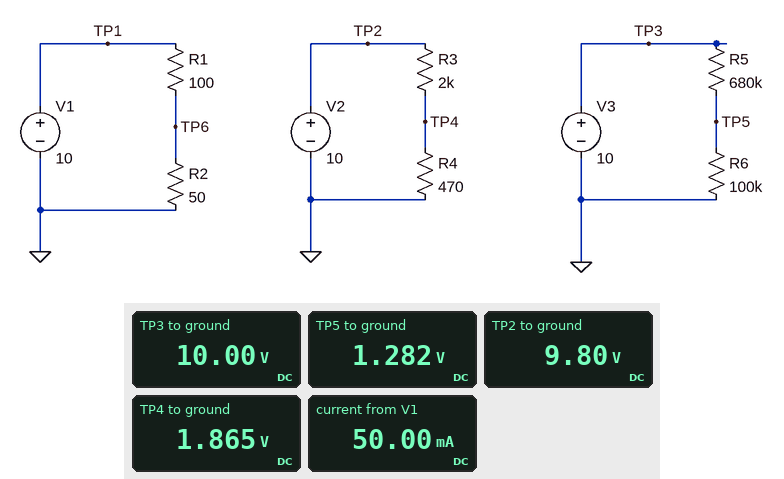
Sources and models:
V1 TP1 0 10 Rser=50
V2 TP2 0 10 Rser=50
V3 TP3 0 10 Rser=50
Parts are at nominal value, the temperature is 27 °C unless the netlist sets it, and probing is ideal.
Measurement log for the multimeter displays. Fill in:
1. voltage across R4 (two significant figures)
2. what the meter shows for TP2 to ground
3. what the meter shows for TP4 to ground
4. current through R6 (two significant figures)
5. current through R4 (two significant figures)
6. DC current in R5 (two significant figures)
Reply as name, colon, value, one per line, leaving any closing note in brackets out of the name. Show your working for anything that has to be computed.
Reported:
voltage across R4: 1.865 V = 1.9 V
what the meter shows for TP2 to ground: 9.80 V
what the meter shows for TP4 to ground: 1.865 V
current through R6: (1.282 V) / 100 kΩ = 13 µA
current through R4: (1.865 V) / 470 Ω = 4.0 mA
DC current in R5: (10 V - 1.282 V) / 680 kΩ = 13 µA
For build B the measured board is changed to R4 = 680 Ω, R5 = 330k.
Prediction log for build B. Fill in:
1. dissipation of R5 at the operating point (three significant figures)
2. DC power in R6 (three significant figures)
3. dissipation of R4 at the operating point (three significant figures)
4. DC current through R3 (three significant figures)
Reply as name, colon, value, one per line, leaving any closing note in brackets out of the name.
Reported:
dissipation of R5 at the operating point: 178 µW
DC power in R6: 54.1 µW
dissipation of R4 at the operating point: 9.12 mW
DC current through R3: 3.66 mA
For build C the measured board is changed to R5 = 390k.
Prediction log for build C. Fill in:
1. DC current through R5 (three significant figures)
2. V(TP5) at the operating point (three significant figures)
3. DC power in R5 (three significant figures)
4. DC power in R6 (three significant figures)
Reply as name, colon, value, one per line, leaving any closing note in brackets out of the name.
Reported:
DC current through R5: 20.4 µA
V(TP5) at the operating point: 2.04 V
DC power in R5: 162 µW
DC power in R6: 41.6 µW
